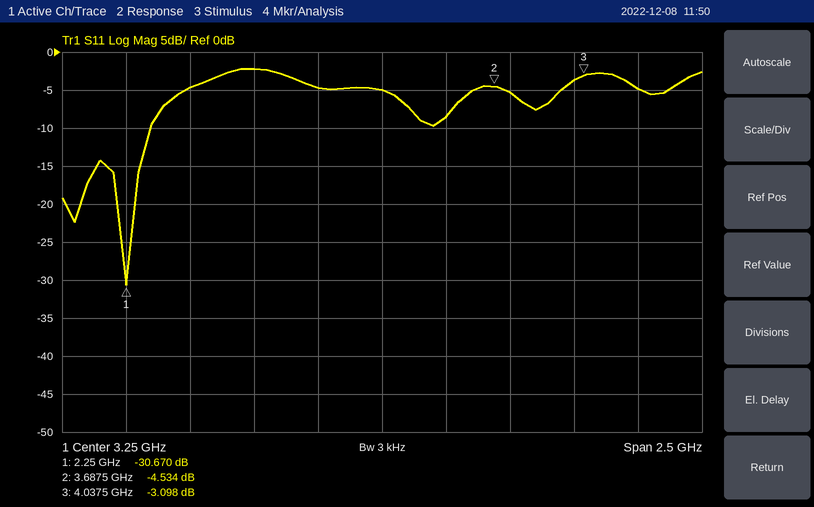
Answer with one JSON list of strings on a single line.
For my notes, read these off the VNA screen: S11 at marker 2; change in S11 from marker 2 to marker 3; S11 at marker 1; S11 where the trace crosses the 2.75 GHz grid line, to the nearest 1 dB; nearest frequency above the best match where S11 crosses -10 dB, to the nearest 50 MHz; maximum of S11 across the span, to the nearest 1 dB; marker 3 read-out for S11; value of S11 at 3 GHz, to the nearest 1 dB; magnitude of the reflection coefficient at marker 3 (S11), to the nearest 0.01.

["-4.534 dB", "1.436 dB", "-30.670 dB", "-2 dB", "2.35 GHz", "-2 dB", "-3.098 dB", "-5 dB", "0.70"]
